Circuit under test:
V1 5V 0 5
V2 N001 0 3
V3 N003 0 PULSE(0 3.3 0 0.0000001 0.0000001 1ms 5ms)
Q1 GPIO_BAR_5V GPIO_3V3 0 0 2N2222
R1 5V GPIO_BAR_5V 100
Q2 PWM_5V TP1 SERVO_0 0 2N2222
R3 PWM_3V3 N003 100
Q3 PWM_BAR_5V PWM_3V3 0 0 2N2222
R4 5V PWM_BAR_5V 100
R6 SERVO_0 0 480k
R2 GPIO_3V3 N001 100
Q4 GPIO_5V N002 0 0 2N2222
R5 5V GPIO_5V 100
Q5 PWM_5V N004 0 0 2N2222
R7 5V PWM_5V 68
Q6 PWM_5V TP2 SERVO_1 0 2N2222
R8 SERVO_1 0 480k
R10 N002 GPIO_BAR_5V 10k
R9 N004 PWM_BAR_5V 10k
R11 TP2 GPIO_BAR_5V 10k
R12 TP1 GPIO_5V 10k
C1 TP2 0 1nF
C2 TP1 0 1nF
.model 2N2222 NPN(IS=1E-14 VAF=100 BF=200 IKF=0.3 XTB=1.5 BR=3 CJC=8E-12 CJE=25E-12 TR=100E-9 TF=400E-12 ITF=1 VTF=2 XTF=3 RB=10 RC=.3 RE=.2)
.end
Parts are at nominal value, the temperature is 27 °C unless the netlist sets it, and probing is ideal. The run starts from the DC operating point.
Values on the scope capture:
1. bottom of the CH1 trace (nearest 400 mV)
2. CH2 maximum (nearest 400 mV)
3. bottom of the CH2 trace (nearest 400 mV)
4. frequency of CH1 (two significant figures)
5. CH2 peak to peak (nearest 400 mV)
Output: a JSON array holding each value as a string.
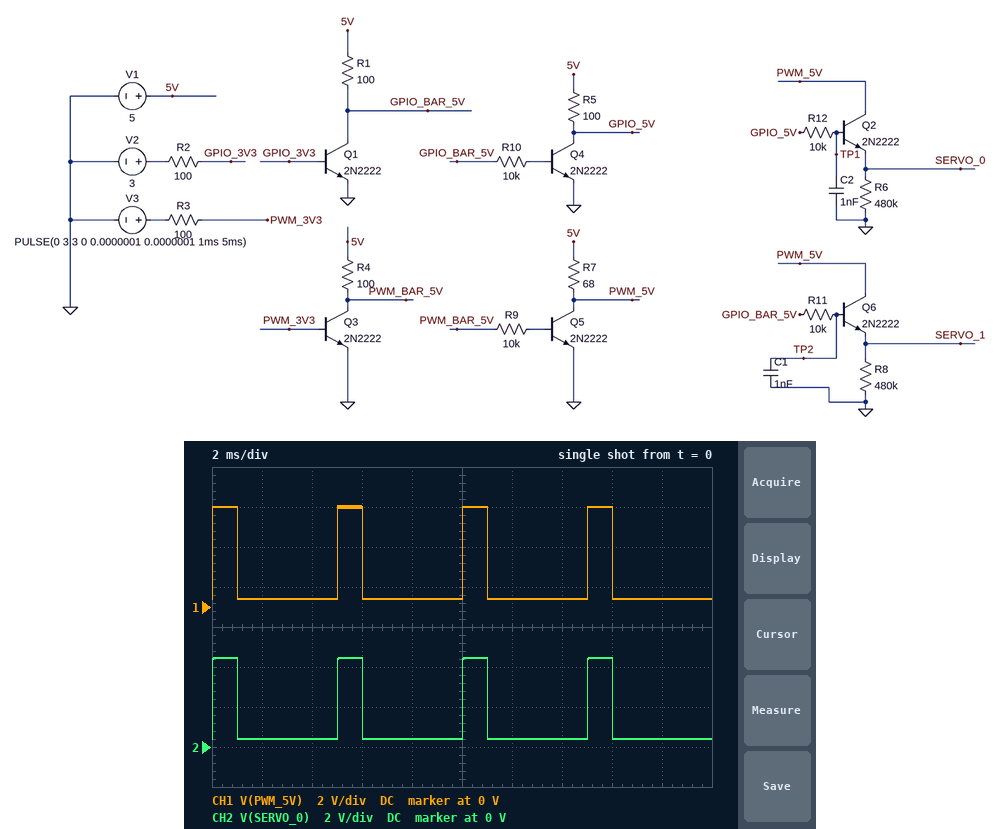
["400 mV", "4.4 V", "400 mV", "200 Hz", "4.0 V"]
